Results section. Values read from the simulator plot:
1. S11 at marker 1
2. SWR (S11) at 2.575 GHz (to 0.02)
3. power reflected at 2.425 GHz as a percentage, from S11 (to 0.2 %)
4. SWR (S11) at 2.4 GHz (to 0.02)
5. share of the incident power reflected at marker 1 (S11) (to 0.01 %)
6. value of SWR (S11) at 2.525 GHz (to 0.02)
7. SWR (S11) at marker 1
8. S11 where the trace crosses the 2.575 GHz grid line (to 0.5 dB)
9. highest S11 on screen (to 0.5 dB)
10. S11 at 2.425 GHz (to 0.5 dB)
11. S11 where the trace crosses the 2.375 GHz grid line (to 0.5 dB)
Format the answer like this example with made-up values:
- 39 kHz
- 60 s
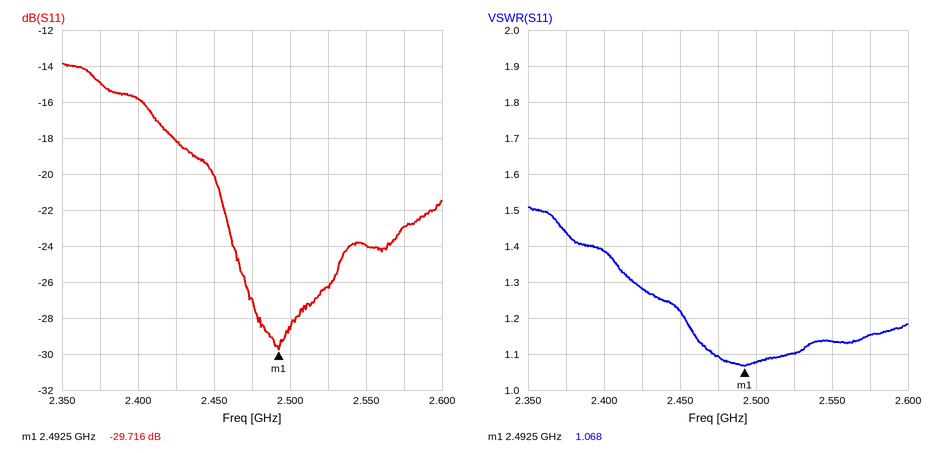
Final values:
- -29.716 dB
- 1.16
- 1.6 %
- 1.38
- 0.11 %
- 1.10
- 1.068
- -23.0 dB
- -14.0 dB
- -18.0 dB
- -15.0 dB
